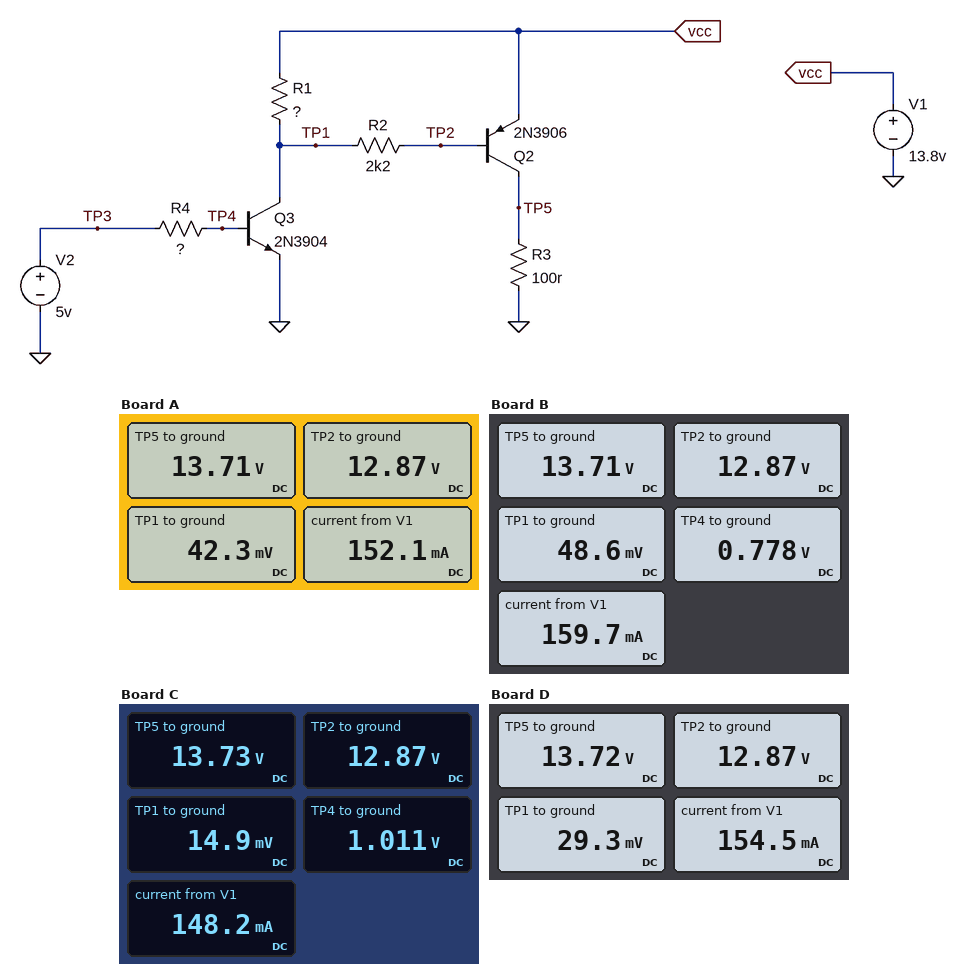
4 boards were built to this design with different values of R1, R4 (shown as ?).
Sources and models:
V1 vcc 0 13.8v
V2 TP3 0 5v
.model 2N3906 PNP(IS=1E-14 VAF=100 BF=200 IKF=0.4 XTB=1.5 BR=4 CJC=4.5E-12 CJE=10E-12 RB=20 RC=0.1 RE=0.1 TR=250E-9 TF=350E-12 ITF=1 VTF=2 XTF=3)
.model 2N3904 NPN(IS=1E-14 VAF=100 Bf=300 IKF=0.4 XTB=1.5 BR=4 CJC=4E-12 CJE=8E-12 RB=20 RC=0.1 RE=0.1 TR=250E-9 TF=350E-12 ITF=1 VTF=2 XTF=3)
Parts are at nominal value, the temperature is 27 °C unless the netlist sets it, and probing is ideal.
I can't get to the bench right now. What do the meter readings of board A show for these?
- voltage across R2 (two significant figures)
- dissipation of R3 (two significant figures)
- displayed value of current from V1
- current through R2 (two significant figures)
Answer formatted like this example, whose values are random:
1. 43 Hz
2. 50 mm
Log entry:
1. 13 V
2. 1.9 W
3. 152.1 mA
4. 5.8 mA
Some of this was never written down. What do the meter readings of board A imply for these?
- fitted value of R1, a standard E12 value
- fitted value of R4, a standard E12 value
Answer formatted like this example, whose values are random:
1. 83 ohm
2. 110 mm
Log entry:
1. 1.5 kΩ
2. 3.3 kΩ
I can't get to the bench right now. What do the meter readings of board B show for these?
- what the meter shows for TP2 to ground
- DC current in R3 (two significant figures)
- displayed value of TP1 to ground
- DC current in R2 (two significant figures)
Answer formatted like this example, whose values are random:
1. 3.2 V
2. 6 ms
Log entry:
1. 12.87 V
2. 140 mA
3. 48.6 mV
4. 5.8 mA
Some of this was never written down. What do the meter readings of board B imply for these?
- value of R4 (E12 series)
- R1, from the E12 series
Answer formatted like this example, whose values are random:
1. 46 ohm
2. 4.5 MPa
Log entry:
1. 2.7 kΩ
2. 820 Ω
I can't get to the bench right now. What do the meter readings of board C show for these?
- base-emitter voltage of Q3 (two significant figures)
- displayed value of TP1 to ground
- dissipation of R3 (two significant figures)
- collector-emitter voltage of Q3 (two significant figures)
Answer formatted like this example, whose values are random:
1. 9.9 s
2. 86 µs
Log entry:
1. 1.0 V
2. 14.9 mV
3. 1.9 W
4. 15 mV
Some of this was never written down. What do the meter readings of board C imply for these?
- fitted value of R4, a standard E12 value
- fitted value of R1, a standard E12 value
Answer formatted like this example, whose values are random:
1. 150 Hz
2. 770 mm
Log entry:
1. 330 Ω
2. 2.7 kΩ
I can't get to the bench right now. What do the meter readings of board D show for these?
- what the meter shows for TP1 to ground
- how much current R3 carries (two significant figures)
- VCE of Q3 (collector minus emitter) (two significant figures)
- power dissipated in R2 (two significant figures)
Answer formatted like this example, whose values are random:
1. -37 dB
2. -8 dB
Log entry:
1. 29.3 mV
2. 140 mA
3. 29 mV
4. 75 mW
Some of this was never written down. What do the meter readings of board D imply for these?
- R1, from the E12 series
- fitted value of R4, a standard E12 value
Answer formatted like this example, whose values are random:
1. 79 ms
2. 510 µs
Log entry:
1. 1.2 kΩ
2. 1.2 kΩ
